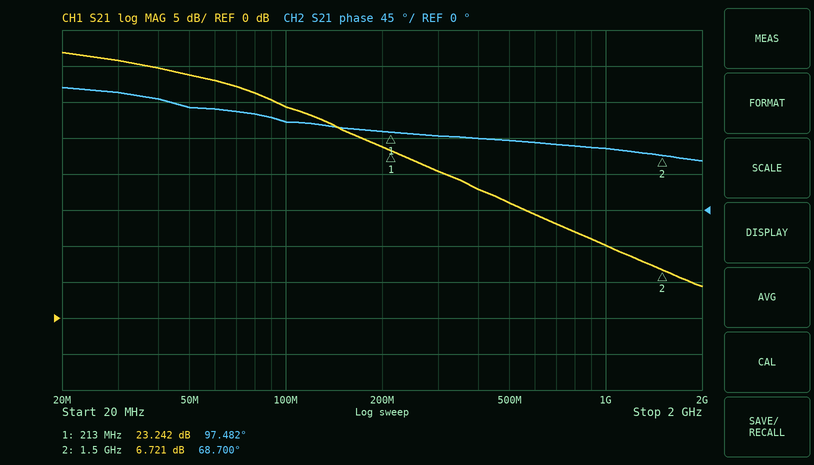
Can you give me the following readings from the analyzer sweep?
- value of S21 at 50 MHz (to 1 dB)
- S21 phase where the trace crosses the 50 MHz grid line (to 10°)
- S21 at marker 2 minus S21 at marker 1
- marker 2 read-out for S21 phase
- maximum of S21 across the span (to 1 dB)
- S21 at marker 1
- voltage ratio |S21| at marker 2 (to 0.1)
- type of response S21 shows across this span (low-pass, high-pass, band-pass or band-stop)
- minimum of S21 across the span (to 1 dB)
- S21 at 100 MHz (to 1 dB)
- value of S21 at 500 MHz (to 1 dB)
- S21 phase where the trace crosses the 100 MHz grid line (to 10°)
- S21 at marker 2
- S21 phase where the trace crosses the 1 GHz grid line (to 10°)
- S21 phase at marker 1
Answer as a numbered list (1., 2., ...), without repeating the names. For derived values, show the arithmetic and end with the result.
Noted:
1. 34 dB
2. 130°
3. 6.721 − (23.242) = -16.521 dB
4. 68.700°
5. 37 dB
6. 23.242 dB
7. 10^(6.721/20) ≈ 2.2
8. low-pass
9. 4 dB
10. 29 dB
11. 16 dB
12. 110°
13. 6.721 dB
14. 80°
15. 97.482°
